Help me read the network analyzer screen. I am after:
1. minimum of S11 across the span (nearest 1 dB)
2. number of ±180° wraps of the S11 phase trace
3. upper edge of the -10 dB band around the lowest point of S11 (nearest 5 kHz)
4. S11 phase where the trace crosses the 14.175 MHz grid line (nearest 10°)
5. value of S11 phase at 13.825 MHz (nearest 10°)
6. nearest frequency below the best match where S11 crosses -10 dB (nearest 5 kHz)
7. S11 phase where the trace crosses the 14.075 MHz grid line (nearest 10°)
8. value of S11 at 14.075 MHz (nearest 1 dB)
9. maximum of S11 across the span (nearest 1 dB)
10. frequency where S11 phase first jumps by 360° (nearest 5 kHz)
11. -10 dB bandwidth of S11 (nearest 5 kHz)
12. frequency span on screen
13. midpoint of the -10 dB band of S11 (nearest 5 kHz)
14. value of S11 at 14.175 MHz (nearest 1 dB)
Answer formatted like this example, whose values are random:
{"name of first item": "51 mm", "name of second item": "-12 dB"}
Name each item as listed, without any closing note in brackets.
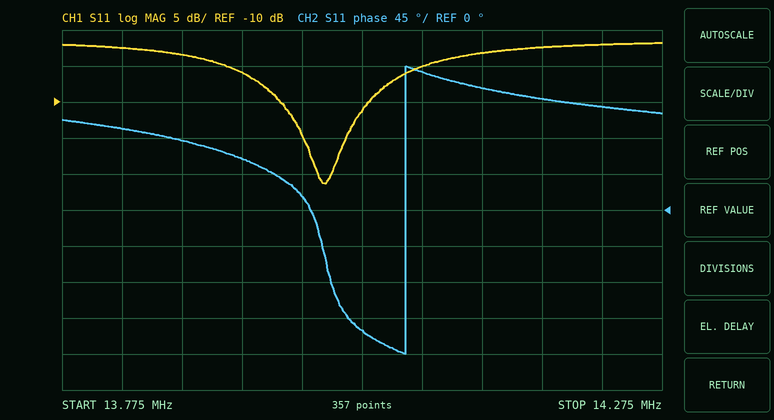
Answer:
{"minimum of S11 across the span": "-21 dB", "number of ±180° wraps of the S11 phase trace": "1", "upper edge of the -10 dB band around the lowest point of S11": "14.030 MHz", "S11 phase where the trace crosses the 14.175 MHz grid line": "140°", "value of S11 phase at 13.825 MHz": "100°", "nearest frequency below the best match where S11 crosses -10 dB": "13.955 MHz", "S11 phase where the trace crosses the 14.075 MHz grid line": "170°", "value of S11 at 14.075 MHz": "-5 dB", "maximum of S11 across the span": "-2 dB", "frequency where S11 phase first jumps by 360°": "14.060 MHz", "-10 dB bandwidth of S11": "75 kHz", "frequency span on screen": "500 kHz", "midpoint of the -10 dB band of S11": "13.995 MHz", "value of S11 at 14.175 MHz": "-2 dB"}
